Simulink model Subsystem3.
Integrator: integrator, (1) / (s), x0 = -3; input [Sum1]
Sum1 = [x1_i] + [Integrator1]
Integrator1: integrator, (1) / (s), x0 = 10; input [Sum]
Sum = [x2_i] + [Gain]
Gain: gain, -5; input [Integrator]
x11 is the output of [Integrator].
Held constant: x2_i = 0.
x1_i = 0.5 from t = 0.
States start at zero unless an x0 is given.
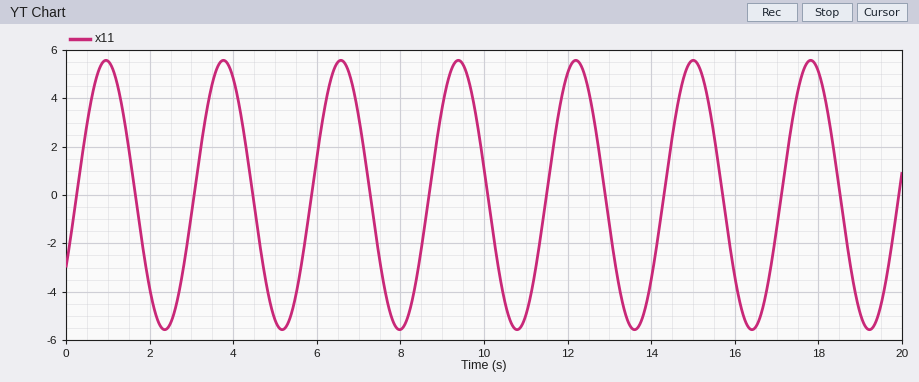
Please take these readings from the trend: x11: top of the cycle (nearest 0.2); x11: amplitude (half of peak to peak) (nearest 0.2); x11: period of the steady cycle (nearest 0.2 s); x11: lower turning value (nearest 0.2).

5.6
5.6
2.8 s
-5.6
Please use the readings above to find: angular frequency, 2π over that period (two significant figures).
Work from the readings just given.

2.2 rad/s
